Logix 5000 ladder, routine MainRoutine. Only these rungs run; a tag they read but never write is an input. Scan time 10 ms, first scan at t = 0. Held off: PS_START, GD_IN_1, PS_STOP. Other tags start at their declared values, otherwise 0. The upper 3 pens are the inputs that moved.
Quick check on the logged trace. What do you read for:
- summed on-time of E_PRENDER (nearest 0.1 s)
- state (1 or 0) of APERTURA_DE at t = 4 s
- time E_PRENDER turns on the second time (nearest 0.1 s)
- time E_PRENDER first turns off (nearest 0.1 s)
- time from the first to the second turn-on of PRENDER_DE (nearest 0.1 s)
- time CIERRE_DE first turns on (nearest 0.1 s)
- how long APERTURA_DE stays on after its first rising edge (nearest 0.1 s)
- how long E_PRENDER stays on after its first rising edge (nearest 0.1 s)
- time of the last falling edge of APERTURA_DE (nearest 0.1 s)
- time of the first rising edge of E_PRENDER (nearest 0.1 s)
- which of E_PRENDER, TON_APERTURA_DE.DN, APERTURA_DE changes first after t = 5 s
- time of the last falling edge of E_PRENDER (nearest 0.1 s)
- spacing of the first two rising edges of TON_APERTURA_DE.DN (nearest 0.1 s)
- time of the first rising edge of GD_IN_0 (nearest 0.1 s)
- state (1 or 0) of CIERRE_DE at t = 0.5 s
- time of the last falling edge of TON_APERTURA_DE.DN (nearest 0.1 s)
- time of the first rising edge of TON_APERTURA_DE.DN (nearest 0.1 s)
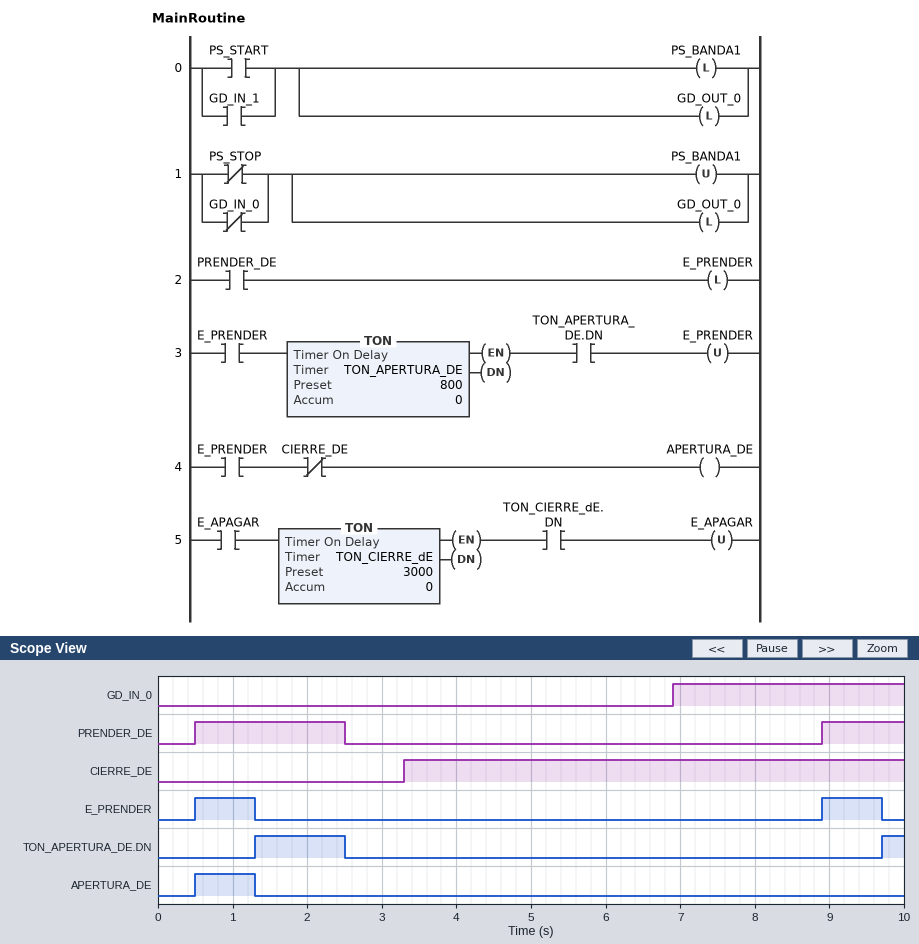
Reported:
1.6 s
0
8.9 s
1.3 s
8.4 s
3.3 s
0.8 s
0.8 s
1.3 s
0.5 s
E_PRENDER
9.7 s
8.4 s
6.9 s
0
2.5 s
1.3 s
